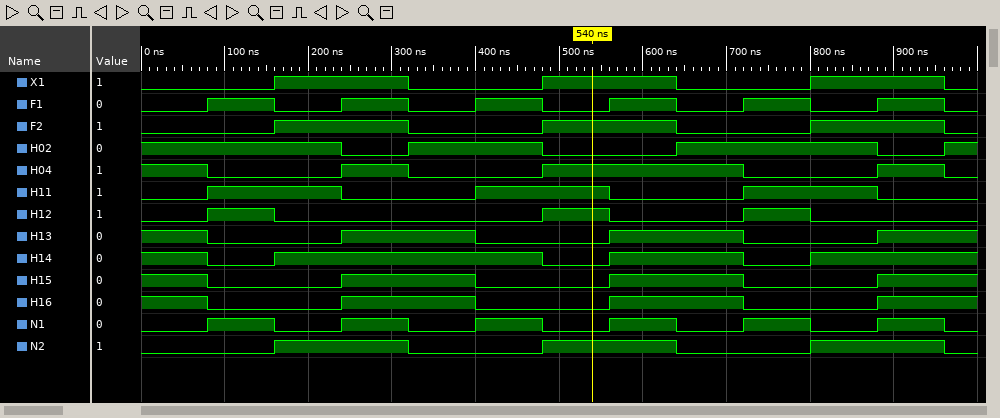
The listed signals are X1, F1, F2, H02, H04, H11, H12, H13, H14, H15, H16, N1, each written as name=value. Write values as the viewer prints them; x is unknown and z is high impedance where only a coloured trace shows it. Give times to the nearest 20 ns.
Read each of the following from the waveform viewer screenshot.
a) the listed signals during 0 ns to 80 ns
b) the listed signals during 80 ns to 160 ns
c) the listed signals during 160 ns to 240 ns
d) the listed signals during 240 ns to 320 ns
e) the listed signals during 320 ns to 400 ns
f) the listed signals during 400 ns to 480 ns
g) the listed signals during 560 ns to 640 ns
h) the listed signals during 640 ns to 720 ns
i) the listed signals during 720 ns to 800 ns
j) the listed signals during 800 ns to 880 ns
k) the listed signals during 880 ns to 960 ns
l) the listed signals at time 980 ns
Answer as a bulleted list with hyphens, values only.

- X1=0, F1=0, F2=0, H02=1, H04=1, H11=0, H12=0, H13=1, H14=1, H15=1, H16=1, N1=0
- X1=0, F1=1, F2=0, H02=1, H04=0, H11=1, H12=1, H13=0, H14=0, H15=0, H16=0, N1=1
- X1=1, F1=0, F2=1, H02=1, H04=0, H11=1, H12=0, H13=0, H14=1, H15=0, H16=0, N1=0
- X1=1, F1=1, F2=1, H02=0, H04=1, H11=0, H12=0, H13=1, H14=1, H15=1, H16=1, N1=1
- X1=0, F1=0, F2=0, H02=1, H04=0, H11=0, H12=0, H13=1, H14=1, H15=1, H16=1, N1=0
- X1=0, F1=1, F2=0, H02=1, H04=0, H11=1, H12=0, H13=0, H14=1, H15=0, H16=0, N1=1
- X1=1, F1=1, F2=1, H02=0, H04=1, H11=0, H12=0, H13=1, H14=1, H15=1, H16=1, N1=1
- X1=0, F1=0, F2=0, H02=1, H04=1, H11=0, H12=0, H13=1, H14=1, H15=1, H16=1, N1=0
- X1=0, F1=1, F2=0, H02=1, H04=0, H11=1, H12=1, H13=0, H14=0, H15=0, H16=0, N1=1
- X1=1, F1=0, F2=1, H02=1, H04=0, H11=1, H12=0, H13=0, H14=1, H15=0, H16=0, N1=0
- X1=1, F1=1, F2=1, H02=0, H04=1, H11=0, H12=0, H13=1, H14=1, H15=1, H16=1, N1=1
- X1=0, F1=0, F2=0, H02=1, H04=0, H11=0, H12=0, H13=1, H14=1, H15=1, H16=1, N1=0
